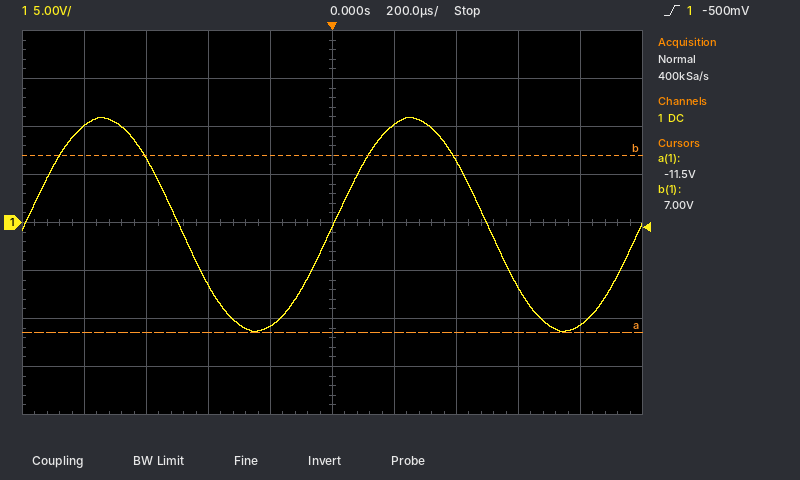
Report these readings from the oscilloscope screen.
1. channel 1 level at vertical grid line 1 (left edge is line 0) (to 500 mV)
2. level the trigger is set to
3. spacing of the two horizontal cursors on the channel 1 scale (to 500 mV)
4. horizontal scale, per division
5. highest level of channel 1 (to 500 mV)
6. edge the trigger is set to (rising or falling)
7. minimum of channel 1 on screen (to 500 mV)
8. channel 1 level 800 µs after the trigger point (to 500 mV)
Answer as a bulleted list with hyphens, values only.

- 10.0 V
- -500 mV
- 18.5 V
- 200 µs
- 11.0 V
- rising
- -11.5 V
- -10.5 V
